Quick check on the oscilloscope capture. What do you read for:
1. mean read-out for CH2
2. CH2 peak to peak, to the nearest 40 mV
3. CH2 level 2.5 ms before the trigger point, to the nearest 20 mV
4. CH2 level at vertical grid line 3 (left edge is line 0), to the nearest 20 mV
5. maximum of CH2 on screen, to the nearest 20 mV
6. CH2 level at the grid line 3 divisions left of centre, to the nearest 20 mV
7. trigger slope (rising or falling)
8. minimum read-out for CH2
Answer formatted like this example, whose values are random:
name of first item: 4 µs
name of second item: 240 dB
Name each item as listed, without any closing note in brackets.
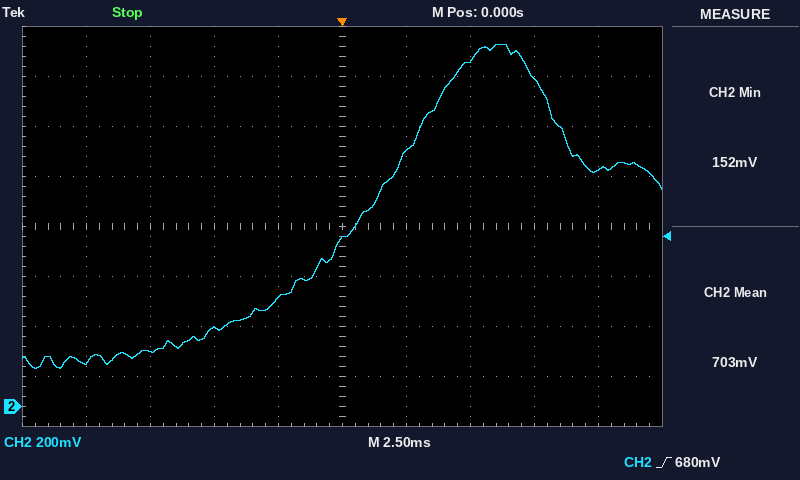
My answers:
mean read-out for CH2: 703 mV
CH2 peak to peak, to the nearest 40 mV: 1.28 V
CH2 level 2.5 ms before the trigger point, to the nearest 20 mV: 440 mV
CH2 level at vertical grid line 3 (left edge is line 0), to the nearest 20 mV: 320 mV
maximum of CH2 on screen, to the nearest 20 mV: 1.44 V
CH2 level at the grid line 3 divisions left of centre, to the nearest 20 mV: 220 mV
trigger slope: rising
minimum read-out for CH2: 152 mV
